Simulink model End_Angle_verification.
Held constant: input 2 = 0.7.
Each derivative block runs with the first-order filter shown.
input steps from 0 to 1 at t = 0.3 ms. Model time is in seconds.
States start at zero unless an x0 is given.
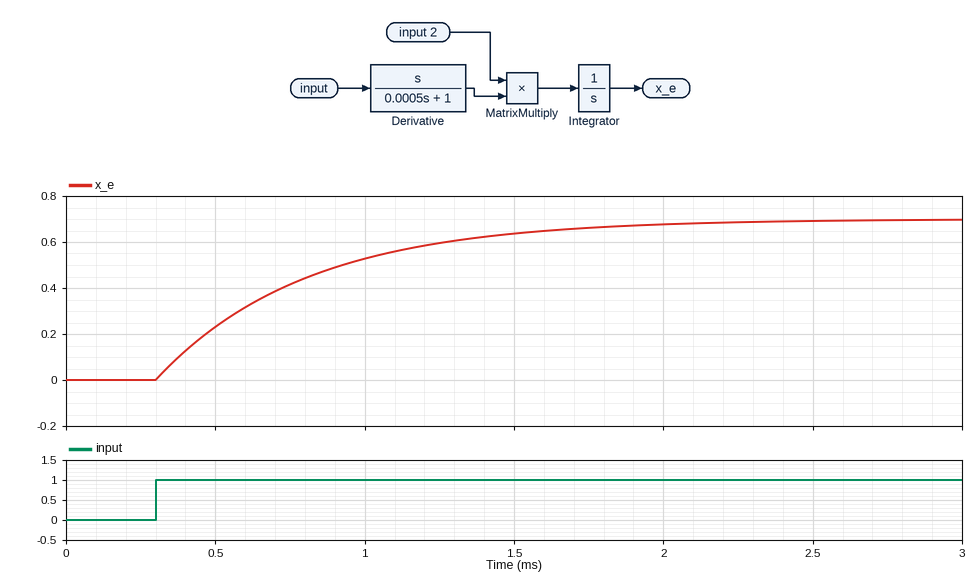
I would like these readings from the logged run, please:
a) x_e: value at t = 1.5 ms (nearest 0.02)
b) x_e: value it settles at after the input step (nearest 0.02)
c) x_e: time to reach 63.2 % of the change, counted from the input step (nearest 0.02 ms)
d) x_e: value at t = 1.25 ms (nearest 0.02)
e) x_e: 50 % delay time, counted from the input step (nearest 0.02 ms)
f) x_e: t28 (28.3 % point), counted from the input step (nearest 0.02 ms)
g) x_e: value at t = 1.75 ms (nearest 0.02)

0.64
0.70
0.50 ms
0.60
0.34 ms
0.16 ms
0.66
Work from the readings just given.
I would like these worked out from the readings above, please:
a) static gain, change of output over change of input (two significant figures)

0.70
